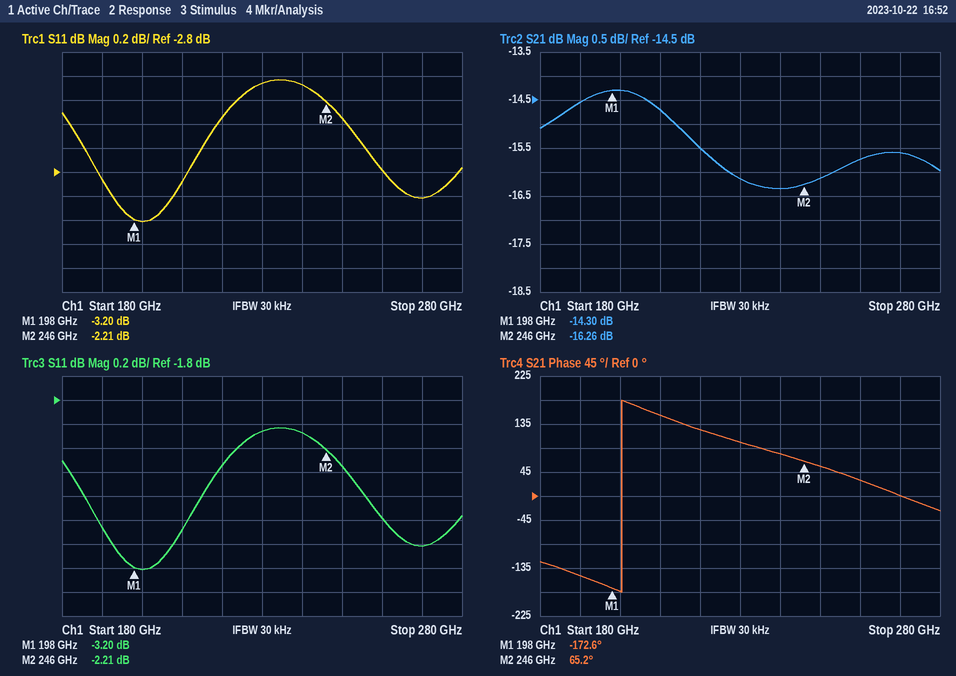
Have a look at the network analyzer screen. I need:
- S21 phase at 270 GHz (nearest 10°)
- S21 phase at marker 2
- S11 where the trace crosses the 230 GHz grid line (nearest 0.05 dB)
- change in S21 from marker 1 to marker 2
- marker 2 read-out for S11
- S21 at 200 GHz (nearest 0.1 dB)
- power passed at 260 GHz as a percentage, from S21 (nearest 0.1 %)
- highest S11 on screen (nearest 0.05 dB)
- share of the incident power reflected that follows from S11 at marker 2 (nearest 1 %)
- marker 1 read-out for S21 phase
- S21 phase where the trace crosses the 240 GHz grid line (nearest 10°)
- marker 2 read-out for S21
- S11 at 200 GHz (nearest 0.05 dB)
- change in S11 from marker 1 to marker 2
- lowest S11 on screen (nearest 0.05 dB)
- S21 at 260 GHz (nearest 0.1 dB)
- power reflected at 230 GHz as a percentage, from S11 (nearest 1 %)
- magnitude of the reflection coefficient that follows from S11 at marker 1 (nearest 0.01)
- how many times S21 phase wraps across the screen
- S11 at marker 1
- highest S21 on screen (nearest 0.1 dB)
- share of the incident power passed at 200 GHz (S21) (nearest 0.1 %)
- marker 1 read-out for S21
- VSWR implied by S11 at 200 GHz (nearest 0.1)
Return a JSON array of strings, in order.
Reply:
["0°", "65.2°", "-2.05 dB", "-1.96 dB", "-2.21 dB", "-14.3 dB", "2.7 %", "-2.05 dB", "60 %", "-172.6°", "80°", "-16.26 dB", "-3.20 dB", "0.99 dB", "-3.20 dB", "-15.7 dB", "62 %", "0.69", "1", "-3.20 dB", "-14.3 dB", "3.7 %", "-14.30 dB", "5.5"]
